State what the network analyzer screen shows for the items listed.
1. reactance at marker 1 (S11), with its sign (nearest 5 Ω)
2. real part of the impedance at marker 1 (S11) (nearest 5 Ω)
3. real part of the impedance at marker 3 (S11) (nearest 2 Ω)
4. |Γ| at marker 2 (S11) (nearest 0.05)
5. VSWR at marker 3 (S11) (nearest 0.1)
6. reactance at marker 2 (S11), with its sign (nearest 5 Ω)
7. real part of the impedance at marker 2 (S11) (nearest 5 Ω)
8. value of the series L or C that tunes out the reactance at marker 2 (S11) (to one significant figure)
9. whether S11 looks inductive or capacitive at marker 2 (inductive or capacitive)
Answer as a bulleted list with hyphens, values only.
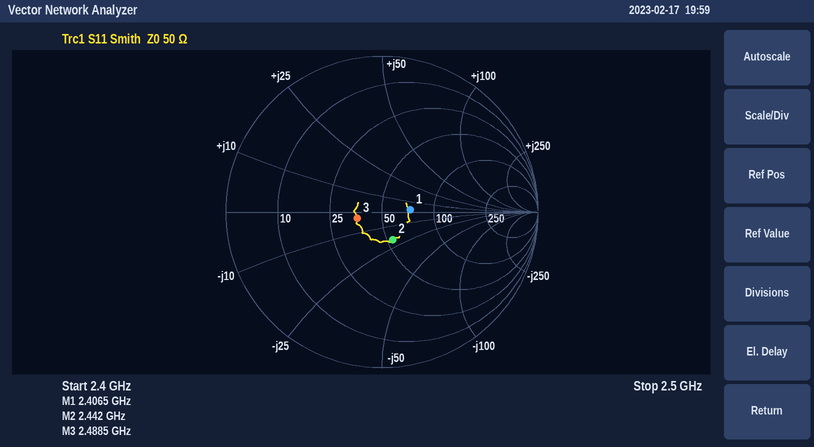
- 0 Ω
- 70 Ω
- 36 Ω
- 0.20
- 1.4
- -20 Ω
- 55 Ω
- 1 nH
- capacitive
